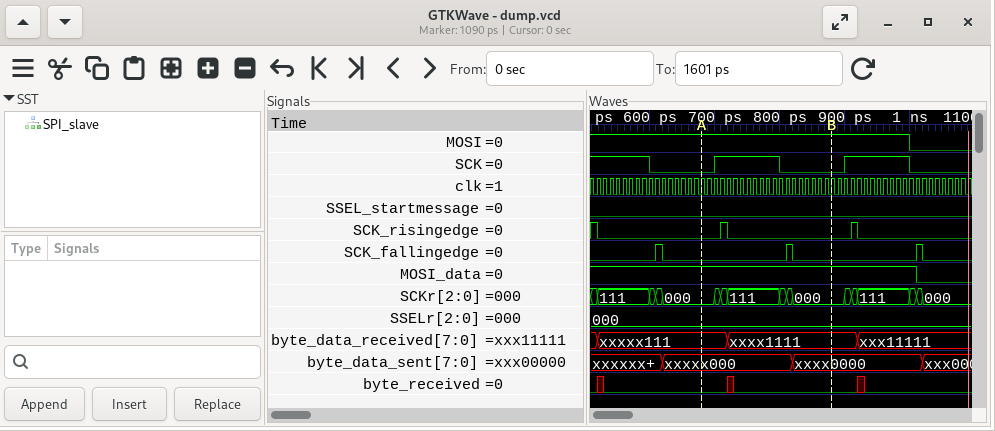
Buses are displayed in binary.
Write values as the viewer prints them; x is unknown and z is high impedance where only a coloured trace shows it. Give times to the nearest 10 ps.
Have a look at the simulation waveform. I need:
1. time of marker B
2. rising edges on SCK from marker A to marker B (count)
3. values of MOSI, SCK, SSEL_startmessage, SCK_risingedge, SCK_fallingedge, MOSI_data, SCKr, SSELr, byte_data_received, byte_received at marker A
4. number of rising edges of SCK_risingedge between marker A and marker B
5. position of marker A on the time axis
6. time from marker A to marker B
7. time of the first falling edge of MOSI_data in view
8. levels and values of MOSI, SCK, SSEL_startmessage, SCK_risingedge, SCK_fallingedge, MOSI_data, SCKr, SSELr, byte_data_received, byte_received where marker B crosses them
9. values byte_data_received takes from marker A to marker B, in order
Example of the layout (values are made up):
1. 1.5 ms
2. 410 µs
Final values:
1. 880 ps
2. 1
3. MOSI=1, SCK=0, SSEL_startmessage=0, SCK_risingedge=0, SCK_fallingedge=0, MOSI_data=1, SCKr=000, SSELr=000, byte_data_received=xxxxx111, byte_received=0
4. 1
5. 680 ps
6. 200 ps
7. 1010 ps
8. MOSI=1, SCK=0, SSEL_startmessage=0, SCK_risingedge=0, SCK_fallingedge=0, MOSI_data=1, SCKr=000, SSELr=000, byte_data_received=xxxx1111, byte_received=0
9. xxxxx111, xxxx1111
